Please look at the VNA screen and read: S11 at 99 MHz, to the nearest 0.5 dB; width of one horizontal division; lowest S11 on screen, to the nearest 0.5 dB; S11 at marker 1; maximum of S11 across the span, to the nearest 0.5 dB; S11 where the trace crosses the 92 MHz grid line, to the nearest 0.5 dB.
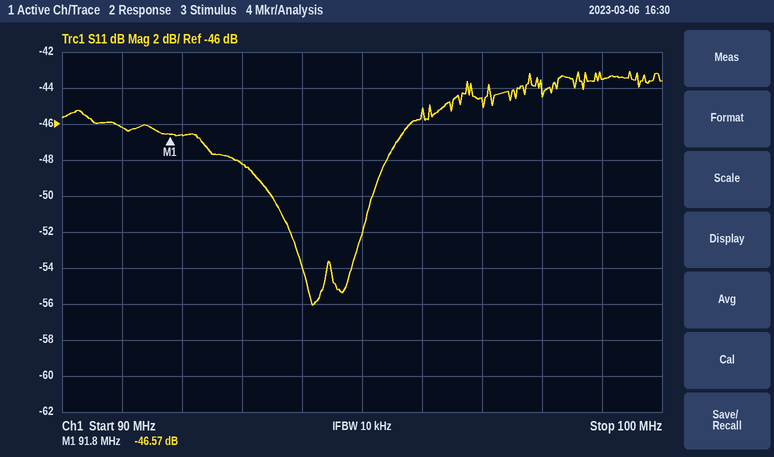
-43.5 dB
1 MHz
-56.0 dB
-46.57 dB
-43.0 dB
-46.5 dB
